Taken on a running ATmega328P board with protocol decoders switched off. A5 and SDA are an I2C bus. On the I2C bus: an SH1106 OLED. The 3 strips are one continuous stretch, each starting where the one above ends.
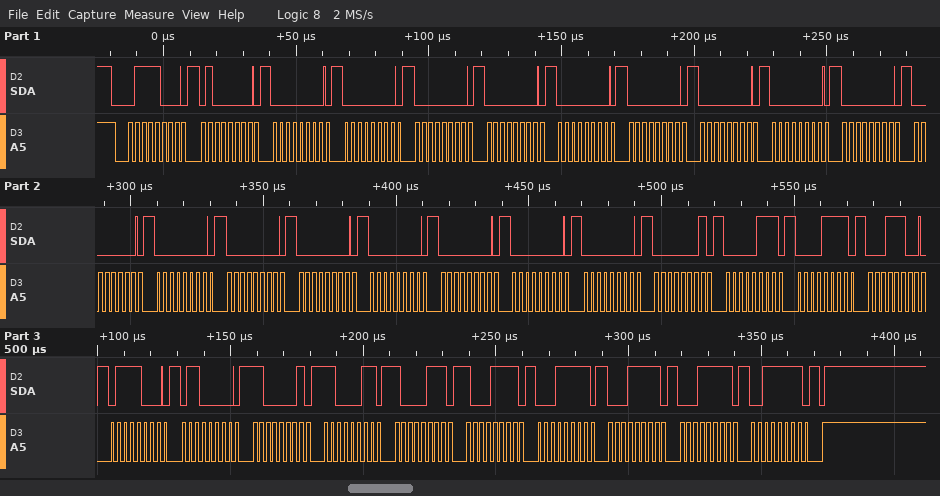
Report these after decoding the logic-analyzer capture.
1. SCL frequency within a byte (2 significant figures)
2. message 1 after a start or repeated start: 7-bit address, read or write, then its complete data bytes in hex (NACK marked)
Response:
400 kHz
0x3C write: 40 00 00 00 00 00 00 00 00 00 00 00 00 00 00 00 00 00 01 07 0F 1C 78 60 C1 C3 87 8F 1F 1F 1F 3F
